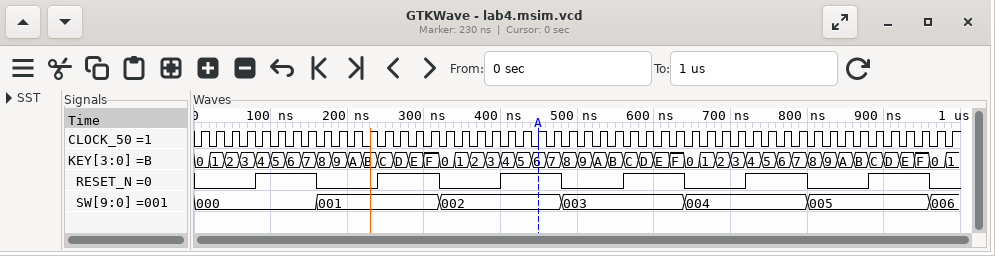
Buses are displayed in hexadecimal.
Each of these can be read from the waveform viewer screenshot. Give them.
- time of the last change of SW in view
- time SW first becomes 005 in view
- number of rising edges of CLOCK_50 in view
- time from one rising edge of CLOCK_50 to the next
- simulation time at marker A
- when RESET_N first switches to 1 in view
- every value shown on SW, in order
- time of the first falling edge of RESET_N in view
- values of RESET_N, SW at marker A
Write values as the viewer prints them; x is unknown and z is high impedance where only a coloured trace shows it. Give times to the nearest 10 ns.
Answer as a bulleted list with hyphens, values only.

- 960 ns
- 800 ns
- 50
- 20 ns
- 450 ns
- 80 ns
- 000, 001, 002, 003, 004, 005, 006
- 160 ns
- RESET_N=1, SW=002
